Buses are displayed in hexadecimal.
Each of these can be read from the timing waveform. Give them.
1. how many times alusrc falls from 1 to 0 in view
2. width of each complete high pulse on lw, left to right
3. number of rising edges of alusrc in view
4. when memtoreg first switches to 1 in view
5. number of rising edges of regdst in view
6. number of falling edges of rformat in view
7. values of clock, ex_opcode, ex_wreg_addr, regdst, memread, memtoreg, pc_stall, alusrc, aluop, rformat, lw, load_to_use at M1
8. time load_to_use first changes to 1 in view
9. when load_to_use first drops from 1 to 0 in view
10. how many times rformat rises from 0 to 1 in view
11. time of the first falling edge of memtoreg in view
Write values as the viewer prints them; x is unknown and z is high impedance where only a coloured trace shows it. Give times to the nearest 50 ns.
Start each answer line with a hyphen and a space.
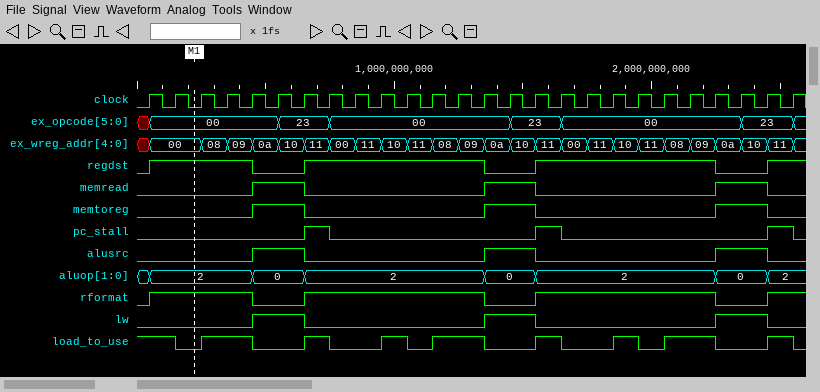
- 3
- 200 ns, 200 ns, 200 ns
- 3
- 450 ns
- 4
- 3
- clock=0, ex_opcode=00, ex_wreg_addr=00, regdst=1, memread=0, memtoreg=0, pc_stall=0, alusrc=0, aluop=2, rformat=1, lw=0, load_to_use=0
- 250 ns
- 150 ns
- 4
- 650 ns
